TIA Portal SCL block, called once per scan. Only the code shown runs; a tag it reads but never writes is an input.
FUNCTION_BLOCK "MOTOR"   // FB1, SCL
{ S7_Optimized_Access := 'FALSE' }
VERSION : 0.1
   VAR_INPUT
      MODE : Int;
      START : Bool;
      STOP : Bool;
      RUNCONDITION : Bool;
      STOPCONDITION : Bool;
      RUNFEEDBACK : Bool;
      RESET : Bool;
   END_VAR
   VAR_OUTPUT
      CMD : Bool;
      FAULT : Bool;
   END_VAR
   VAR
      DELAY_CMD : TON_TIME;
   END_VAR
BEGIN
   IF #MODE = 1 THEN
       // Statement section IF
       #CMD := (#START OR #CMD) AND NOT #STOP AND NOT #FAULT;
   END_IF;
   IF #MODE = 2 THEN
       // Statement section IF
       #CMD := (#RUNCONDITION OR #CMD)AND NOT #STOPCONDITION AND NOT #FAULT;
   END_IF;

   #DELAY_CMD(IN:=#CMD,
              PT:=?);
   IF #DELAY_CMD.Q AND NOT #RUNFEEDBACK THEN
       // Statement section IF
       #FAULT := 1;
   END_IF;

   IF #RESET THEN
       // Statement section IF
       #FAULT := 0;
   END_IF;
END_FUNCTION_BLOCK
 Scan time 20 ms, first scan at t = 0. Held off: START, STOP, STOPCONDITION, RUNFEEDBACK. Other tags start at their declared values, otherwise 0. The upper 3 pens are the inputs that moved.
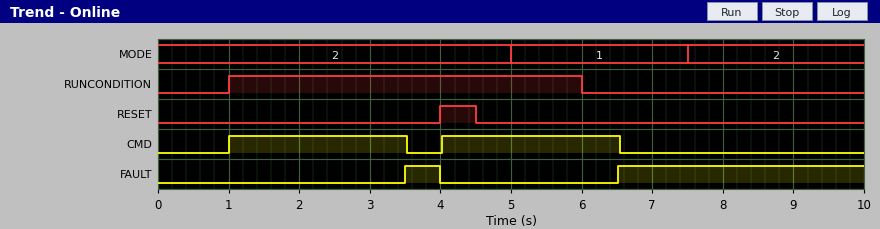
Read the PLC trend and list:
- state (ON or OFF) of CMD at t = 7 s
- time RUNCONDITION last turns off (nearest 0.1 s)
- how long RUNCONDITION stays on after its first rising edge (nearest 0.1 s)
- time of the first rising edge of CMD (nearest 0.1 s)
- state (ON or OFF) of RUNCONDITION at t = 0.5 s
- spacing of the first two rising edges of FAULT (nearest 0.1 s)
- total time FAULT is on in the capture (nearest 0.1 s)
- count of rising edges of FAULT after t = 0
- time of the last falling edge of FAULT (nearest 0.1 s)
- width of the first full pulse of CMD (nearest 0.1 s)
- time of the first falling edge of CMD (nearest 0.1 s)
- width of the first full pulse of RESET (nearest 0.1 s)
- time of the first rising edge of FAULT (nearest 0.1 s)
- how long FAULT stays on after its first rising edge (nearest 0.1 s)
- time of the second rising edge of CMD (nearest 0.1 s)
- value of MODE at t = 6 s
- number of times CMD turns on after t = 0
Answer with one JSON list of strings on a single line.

["OFF", "6.0 s", "5.0 s", "1.0 s", "OFF", "3.0 s", "4.0 s", "2", "4.0 s", "2.5 s", "3.5 s", "0.5 s", "3.5 s", "0.5 s", "4.0 s", "1", "2"]
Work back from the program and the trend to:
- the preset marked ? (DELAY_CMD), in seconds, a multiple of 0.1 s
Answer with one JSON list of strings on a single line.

["2.5 s"]
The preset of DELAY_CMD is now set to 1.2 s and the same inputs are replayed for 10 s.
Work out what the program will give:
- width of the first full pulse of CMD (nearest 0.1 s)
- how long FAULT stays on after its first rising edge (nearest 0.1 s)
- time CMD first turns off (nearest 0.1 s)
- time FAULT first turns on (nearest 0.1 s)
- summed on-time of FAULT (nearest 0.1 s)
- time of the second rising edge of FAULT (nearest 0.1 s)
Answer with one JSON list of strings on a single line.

["1.2 s", "1.8 s", "2.2 s", "2.2 s", "6.6 s", "5.2 s"]
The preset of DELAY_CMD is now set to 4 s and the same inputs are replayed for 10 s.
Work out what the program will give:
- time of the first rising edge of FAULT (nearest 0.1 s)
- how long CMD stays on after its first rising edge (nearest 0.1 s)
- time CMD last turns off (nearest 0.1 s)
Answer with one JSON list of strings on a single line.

["5.0 s", "4.0 s", "5.0 s"]
